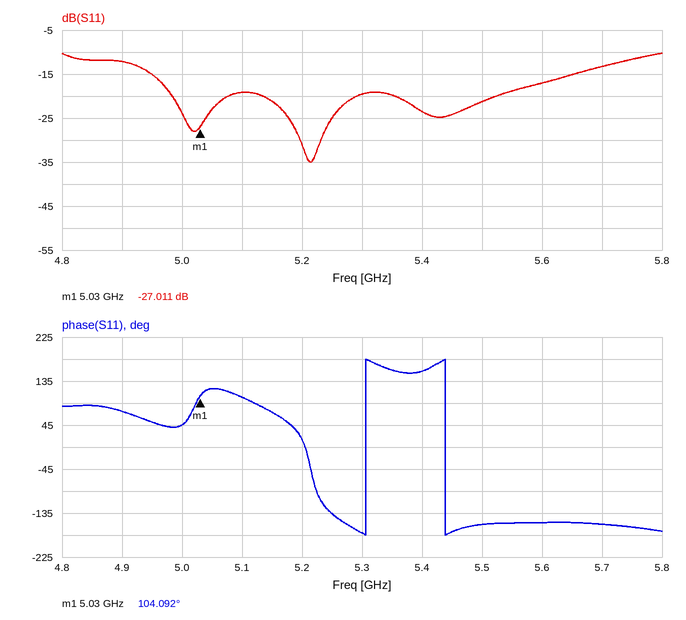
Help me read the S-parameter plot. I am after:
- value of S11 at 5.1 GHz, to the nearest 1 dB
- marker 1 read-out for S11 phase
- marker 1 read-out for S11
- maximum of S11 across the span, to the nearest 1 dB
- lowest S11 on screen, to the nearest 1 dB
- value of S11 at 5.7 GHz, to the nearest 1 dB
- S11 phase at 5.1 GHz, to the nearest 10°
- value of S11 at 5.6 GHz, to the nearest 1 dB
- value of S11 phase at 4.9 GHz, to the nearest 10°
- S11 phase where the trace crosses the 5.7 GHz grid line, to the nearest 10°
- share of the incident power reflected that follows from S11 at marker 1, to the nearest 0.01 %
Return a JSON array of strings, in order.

["-19 dB", "104.092°", "-27.011 dB", "-10 dB", "-35 dB", "-13 dB", "100°", "-17 dB", "70°", "-160°", "0.20 %"]
